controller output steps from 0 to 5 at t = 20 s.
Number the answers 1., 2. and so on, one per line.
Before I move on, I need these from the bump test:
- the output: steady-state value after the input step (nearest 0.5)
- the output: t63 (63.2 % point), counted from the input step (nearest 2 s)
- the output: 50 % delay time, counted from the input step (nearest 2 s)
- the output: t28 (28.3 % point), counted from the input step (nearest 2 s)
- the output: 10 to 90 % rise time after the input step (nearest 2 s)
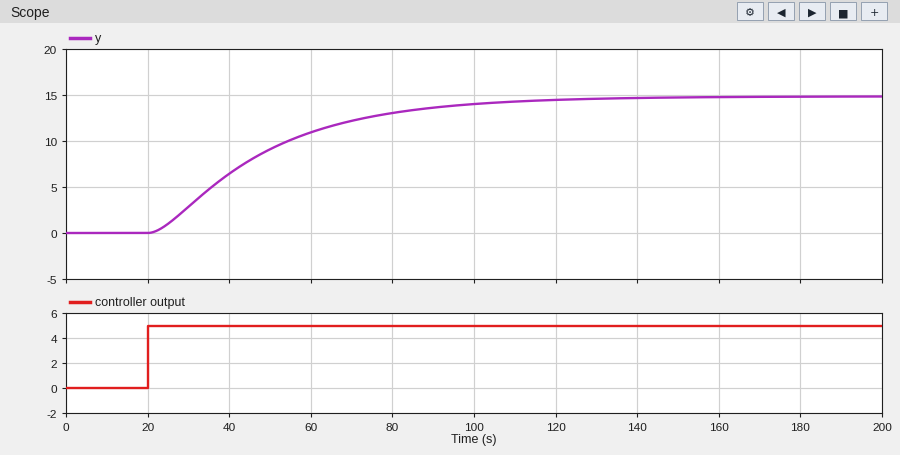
1. 15.0
2. 32 s
3. 24 s
4. 14 s
5. 58 s
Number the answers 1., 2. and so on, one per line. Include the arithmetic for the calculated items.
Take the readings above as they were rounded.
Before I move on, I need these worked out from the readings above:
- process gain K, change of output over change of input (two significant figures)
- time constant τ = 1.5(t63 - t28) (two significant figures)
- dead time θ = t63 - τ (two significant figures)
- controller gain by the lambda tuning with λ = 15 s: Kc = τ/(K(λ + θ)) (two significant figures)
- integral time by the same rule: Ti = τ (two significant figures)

1. (15 - 0) / 5 = 3.0
2. 1.5 × (32 - 14) = 27 s
3. 32 - 27 = 5.0 s
4. 27 / (3 × (15 + 5)) = 0.45
5. 27 s
